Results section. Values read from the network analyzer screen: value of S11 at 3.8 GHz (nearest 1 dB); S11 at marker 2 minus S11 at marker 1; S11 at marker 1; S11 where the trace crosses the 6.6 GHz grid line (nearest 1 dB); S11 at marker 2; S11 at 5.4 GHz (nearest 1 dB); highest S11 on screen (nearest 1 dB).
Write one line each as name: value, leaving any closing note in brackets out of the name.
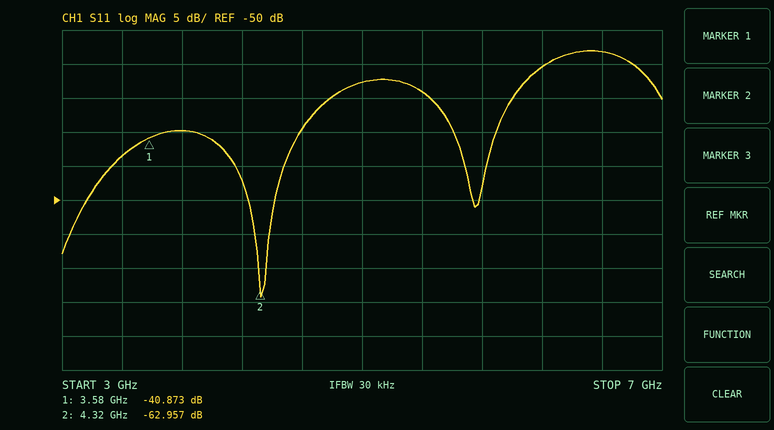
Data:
value of S11 at 3.8 GHz: -40 dB
S11 at marker 2 minus S11 at marker 1: -22.084 dB
S11 at marker 1: -40.873 dB
S11 where the trace crosses the 6.6 GHz grid line: -28 dB
S11 at marker 2: -62.957 dB
S11 at 5.4 GHz: -34 dB
highest S11 on screen: -28 dB
